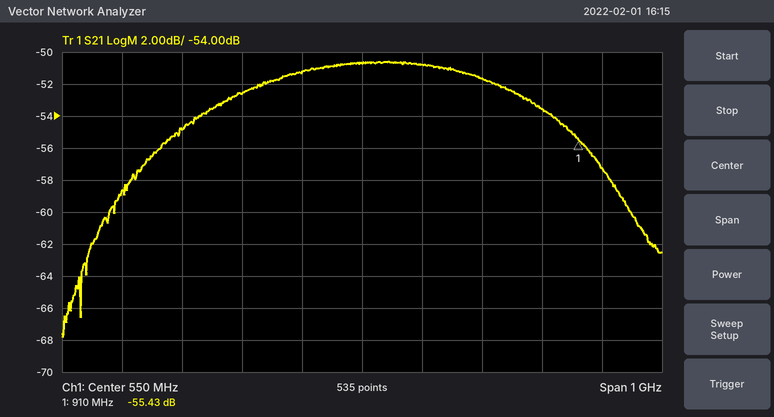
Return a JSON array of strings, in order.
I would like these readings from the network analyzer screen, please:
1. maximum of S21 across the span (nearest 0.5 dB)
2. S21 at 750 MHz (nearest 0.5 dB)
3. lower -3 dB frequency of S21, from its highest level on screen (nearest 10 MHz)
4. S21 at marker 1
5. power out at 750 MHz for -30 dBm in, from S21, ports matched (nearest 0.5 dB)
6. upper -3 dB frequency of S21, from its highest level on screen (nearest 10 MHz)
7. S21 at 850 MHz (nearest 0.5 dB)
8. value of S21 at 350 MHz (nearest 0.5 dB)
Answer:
["-50.5 dB", "-51.5 dB", "300 MHz", "-55.43 dB", "-81.5 dBm", "850 MHz", "-53.5 dB", "-52.5 dB"]
